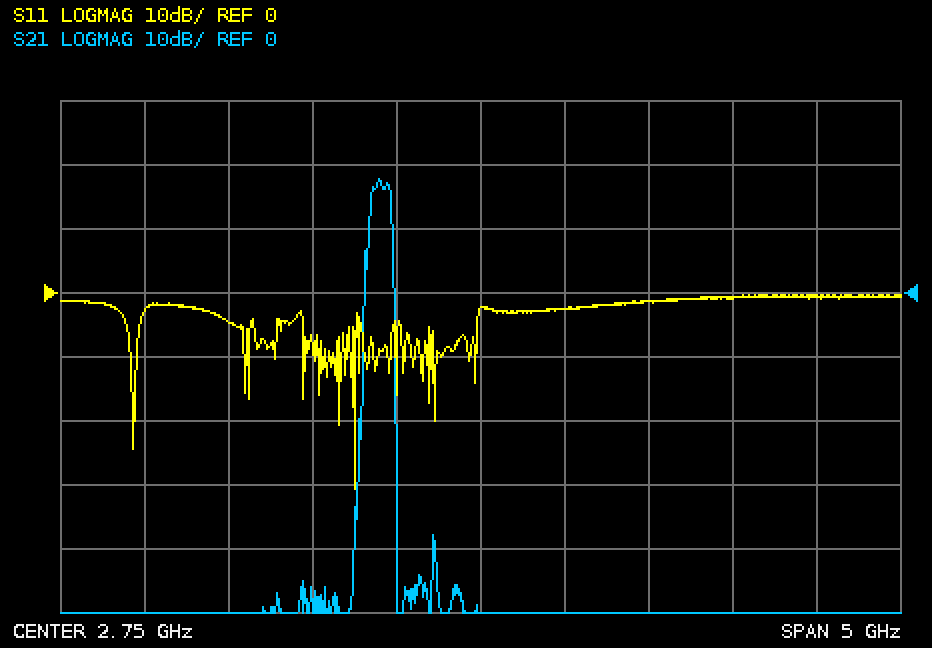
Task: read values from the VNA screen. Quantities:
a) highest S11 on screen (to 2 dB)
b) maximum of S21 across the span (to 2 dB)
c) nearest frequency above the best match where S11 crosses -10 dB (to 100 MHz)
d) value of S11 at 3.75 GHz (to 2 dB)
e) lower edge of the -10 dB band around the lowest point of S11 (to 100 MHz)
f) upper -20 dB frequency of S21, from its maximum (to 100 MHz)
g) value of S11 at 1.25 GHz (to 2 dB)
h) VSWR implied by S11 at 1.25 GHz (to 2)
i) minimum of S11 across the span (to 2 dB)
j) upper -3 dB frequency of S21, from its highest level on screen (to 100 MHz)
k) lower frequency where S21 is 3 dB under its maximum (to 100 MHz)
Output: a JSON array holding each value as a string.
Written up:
["0 dB", "18 dB", "2.0 GHz", "-2 dB", "2.0 GHz", "2.2 GHz", "-4 dB", "4", "-30 dB", "2.2 GHz", "2.1 GHz"]
